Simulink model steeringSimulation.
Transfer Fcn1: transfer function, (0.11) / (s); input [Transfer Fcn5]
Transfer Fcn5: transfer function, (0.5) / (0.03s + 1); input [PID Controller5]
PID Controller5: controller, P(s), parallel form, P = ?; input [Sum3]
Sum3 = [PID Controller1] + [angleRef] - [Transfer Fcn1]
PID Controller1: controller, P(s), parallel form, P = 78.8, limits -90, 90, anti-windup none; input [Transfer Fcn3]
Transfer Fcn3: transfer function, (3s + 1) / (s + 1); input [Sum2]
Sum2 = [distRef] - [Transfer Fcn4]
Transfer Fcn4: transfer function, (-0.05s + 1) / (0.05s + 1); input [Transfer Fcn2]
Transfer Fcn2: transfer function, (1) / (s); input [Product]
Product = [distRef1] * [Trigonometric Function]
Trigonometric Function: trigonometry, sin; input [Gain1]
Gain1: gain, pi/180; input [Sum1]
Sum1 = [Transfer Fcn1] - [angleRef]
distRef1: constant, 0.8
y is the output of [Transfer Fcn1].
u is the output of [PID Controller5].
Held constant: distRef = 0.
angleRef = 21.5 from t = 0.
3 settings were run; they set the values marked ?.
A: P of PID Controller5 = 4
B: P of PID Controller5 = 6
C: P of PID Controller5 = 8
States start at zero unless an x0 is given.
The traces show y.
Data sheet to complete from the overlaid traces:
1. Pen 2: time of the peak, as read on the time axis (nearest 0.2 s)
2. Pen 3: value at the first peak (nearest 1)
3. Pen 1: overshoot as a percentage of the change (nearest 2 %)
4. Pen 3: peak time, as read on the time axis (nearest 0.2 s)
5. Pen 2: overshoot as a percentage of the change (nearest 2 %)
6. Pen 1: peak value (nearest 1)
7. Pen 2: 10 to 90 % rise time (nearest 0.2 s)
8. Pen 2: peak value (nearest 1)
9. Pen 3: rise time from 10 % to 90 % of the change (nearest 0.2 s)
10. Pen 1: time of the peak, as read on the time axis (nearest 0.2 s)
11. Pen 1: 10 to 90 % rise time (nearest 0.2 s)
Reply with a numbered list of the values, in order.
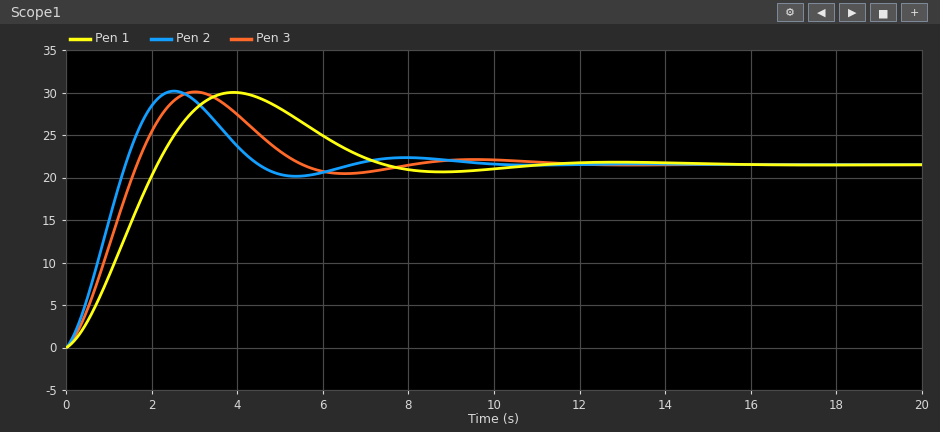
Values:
1. 2.6 s
2. 30
3. 40 %
4. 3.0 s
5. 40 %
6. 30
7. 1.0 s
8. 30
9. 1.2 s
10. 4.0 s
11. 1.6 s
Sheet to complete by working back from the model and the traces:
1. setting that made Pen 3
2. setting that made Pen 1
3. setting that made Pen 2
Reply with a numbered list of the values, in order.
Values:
1. B
2. A
3. C
